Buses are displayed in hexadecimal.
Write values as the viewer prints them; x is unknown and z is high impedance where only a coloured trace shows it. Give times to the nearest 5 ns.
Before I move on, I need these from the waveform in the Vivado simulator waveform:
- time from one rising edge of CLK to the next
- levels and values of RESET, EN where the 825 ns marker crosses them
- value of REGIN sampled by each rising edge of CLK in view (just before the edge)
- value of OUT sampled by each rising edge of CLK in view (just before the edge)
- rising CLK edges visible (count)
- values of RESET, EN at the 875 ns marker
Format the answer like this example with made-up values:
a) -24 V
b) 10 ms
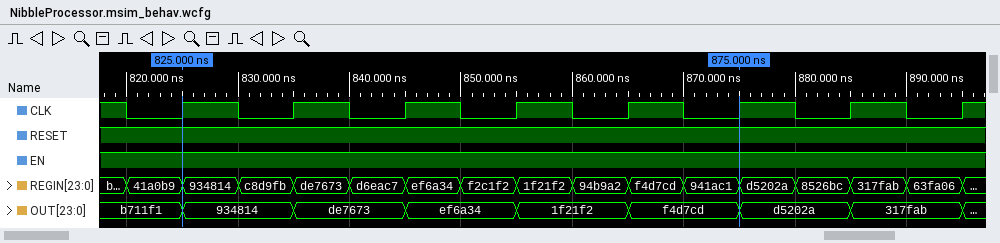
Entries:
a) 10 ns
b) RESET=1, EN=1
c) 41a0b9, c8d9fb, d6eac7, f2c1f2, 94b9a2, 941ac1, 8526bc, 63fa06
d) b711f1, 934814, de7673, ef6a34, 1f21f2, f4d7cd, d5202a, 317fab
e) 8
f) RESET=1, EN=1
